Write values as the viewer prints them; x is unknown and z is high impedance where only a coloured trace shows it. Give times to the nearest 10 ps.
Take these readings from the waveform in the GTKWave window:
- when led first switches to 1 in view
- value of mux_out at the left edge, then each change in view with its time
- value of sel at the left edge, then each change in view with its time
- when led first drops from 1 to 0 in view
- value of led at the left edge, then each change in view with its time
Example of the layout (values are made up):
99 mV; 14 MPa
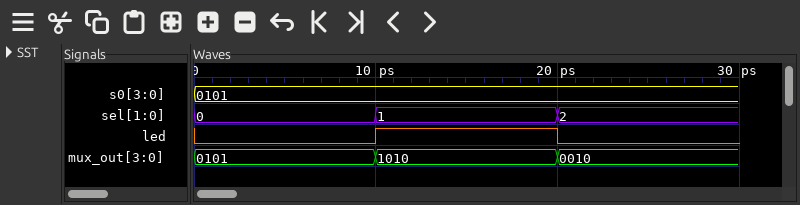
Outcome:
10 ps; 0101, 1010 at 10 ps, 0010 at 20 ps; 0, 1 at 10 ps, 2 at 20 ps; 20 ps; 0, 1 at 10 ps, 0 at 20 ps
